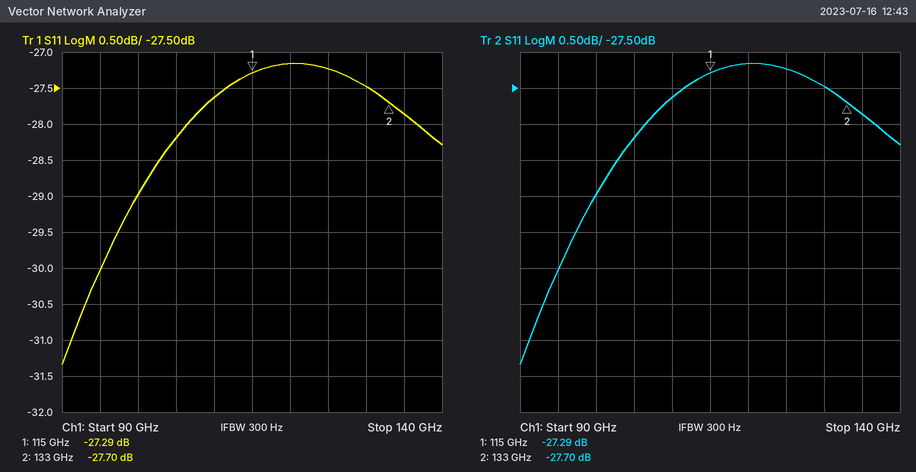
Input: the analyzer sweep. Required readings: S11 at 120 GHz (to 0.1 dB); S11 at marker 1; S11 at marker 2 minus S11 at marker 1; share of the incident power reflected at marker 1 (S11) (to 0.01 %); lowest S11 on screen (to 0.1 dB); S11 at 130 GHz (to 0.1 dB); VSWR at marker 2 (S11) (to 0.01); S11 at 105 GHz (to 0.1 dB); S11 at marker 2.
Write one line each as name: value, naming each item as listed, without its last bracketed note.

S11 at 120 GHz: -27.2 dB
S11 at marker 1: -27.29 dB
S11 at marker 2 minus S11 at marker 1: -0.41 dB
share of the incident power reflected at marker 1 (S11): 0.19 %
lowest S11 on screen: -31.3 dB
S11 at 130 GHz: -27.5 dB
VSWR at marker 2 (S11): 1.09
S11 at 105 GHz: -28.2 dB
S11 at marker 2: -27.70 dB
